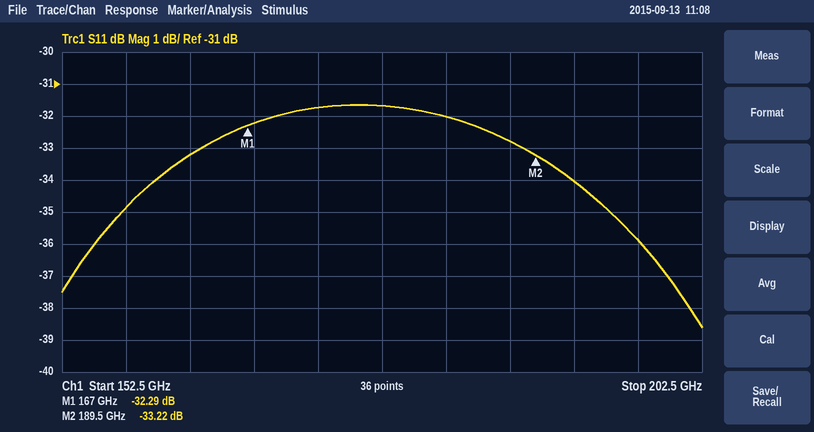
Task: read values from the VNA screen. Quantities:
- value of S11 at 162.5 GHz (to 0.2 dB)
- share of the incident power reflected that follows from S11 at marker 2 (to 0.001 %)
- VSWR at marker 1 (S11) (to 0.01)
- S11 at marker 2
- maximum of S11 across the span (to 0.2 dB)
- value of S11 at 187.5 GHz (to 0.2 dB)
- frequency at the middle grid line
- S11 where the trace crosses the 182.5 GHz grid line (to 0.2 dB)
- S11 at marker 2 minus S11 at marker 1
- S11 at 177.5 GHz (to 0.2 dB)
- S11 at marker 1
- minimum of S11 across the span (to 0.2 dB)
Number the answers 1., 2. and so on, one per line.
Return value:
1. -33.2 dB
2. 0.048 %
3. 1.05
4. -33.22 dB
5. -31.6 dB
6. -32.8 dB
7. 177.5 GHz
8. -32.0 dB
9. -0.93 dB
10. -31.6 dB
11. -32.29 dB
12. -38.6 dB
